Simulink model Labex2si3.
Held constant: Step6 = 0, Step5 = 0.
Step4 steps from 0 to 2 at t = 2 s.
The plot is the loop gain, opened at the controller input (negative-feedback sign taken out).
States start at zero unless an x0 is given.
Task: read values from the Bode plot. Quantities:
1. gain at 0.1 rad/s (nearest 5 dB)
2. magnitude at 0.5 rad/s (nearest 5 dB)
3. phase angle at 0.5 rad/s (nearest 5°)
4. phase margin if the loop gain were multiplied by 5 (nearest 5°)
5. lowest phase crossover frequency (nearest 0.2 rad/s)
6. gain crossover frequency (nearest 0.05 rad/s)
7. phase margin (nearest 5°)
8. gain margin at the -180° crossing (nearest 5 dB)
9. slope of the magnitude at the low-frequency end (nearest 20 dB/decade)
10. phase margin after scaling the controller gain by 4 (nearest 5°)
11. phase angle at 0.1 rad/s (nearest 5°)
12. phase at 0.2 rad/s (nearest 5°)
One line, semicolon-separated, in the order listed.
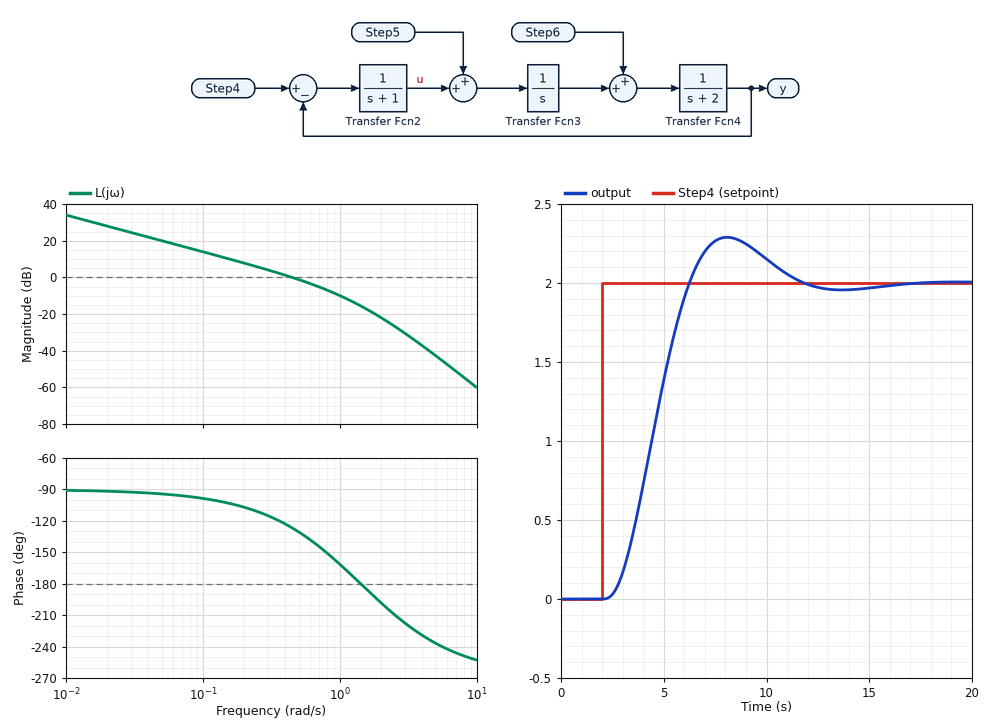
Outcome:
15 dB; 0 dB; -130°; 5°; 1.4 rad/s; 0.45 rad/s; 55°; 15 dB; -20 dB/decade; 10°; -100°; -105°
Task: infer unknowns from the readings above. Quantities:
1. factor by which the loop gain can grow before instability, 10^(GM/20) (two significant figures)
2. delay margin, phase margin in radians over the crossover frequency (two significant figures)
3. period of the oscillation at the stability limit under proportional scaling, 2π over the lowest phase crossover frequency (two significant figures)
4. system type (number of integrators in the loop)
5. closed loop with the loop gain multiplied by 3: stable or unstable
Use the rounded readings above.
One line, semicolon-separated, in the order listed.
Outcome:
5.6; 2.1 s; 4.5 s; 1; stable
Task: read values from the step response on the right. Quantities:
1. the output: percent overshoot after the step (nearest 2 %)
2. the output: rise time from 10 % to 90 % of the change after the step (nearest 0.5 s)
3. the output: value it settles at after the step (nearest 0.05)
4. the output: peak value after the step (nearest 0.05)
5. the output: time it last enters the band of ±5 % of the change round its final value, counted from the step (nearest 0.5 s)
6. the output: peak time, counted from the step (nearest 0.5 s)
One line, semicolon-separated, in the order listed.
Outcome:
14 %; 2.5 s; 2.00; 2.30; 8.5 s; 6.0 s
